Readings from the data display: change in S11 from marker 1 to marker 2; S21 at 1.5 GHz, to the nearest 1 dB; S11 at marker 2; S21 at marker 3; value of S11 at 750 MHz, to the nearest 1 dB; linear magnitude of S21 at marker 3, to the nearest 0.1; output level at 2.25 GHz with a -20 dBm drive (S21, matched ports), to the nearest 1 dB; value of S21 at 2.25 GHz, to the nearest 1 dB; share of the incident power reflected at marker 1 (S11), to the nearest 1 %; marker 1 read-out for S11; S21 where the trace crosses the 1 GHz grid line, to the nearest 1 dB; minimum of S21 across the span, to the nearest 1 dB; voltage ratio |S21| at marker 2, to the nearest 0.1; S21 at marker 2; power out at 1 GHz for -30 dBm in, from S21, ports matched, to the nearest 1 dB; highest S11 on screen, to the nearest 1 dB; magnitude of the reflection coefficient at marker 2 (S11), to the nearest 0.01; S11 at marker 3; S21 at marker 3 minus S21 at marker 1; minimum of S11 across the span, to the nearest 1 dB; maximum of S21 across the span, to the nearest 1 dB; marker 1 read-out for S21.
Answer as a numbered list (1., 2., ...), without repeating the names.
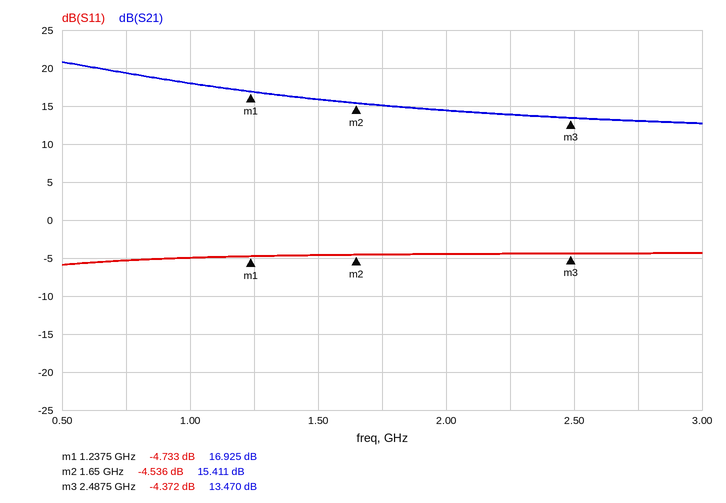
1. 0.197 dB
2. 16 dB
3. -4.536 dB
4. 13.470 dB
5. -5 dB
6. 4.7
7. -6 dBm
8. 14 dB
9. 34 %
10. -4.733 dB
11. 18 dB
12. 13 dB
13. 5.9
14. 15.411 dB
15. -12 dBm
16. -4 dB
17. 0.59
18. -4.372 dB
19. -3.455 dB
20. -6 dB
21. 21 dB
22. 16.925 dB
